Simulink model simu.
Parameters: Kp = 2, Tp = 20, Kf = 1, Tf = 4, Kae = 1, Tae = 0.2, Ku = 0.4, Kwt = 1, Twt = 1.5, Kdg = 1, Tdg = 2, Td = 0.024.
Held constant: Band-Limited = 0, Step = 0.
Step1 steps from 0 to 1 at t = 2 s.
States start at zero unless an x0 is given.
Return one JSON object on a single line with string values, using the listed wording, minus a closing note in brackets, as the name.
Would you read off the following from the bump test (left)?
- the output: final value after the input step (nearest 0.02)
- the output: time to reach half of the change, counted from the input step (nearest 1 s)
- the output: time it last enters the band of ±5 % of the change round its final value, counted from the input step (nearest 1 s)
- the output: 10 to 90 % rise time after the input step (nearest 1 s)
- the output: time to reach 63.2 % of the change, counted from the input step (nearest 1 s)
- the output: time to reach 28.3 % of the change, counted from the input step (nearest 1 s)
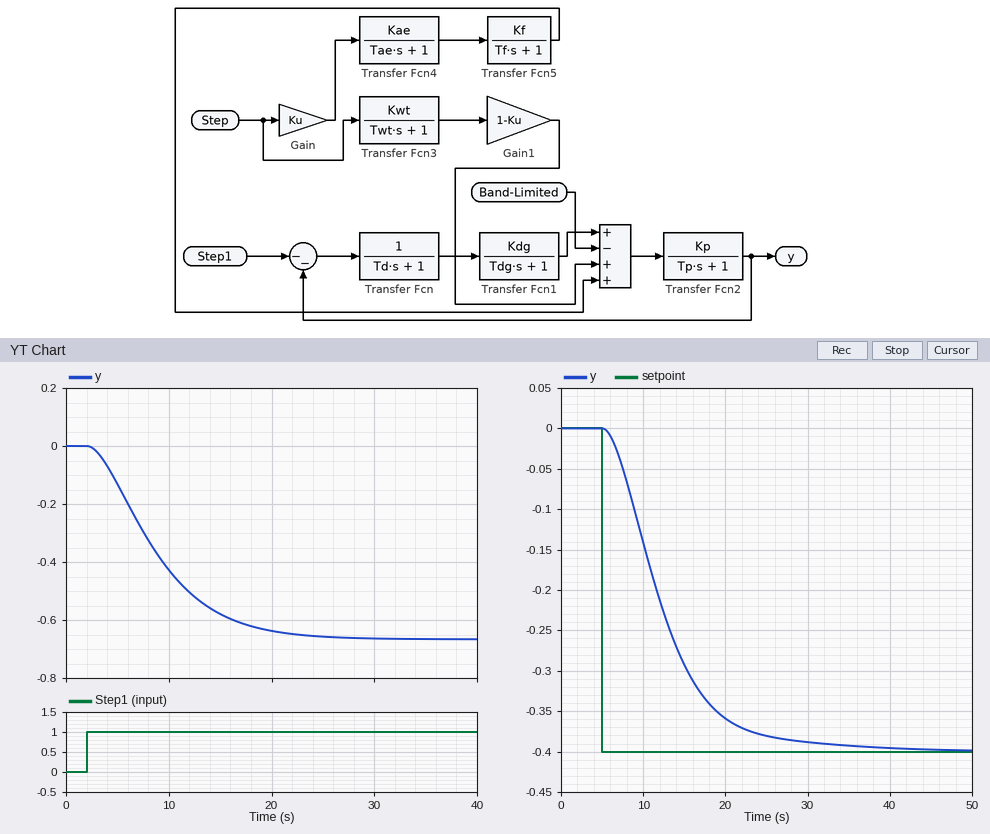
{"the output: final value after the input step": "-0.66", "the output: time to reach half of the change, counted from the input step": "6 s", "the output: time it last enters the band of ±5 % of the change round its final value, counted from the input step": "17 s", "the output: 10 to 90 % rise time after the input step": "12 s", "the output: time to reach 63.2 % of the change, counted from the input step": "8 s", "the output: time to reach 28.3 % of the change, counted from the input step": "4 s"}
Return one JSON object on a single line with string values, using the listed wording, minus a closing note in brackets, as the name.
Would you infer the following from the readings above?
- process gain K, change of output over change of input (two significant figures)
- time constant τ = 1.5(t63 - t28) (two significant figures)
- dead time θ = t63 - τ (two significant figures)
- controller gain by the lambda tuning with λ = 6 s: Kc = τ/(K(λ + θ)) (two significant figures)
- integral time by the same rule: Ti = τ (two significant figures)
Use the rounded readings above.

{"process gain K, change of output over change of input": "-0.66", "time constant τ = 1.5(t63 - t28)": "6.0 s", "dead time θ = t63 - τ": "2.0 s", "controller gain by the lambda tuning with λ = 6 s: Kc = τ/(K(λ + θ))": "-1.1", "integral time by the same rule: Ti = τ": "6.0 s"}
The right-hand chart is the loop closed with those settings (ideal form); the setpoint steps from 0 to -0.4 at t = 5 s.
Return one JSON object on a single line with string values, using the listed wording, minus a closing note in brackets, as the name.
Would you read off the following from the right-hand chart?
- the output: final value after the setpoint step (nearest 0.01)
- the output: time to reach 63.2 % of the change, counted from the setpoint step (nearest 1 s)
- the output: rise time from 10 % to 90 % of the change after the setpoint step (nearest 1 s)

{"the output: final value after the setpoint step": "-0.40", "the output: time to reach 63.2 % of the change, counted from the setpoint step": "8 s", "the output: rise time from 10 % to 90 % of the change after the setpoint step": "13 s"}
